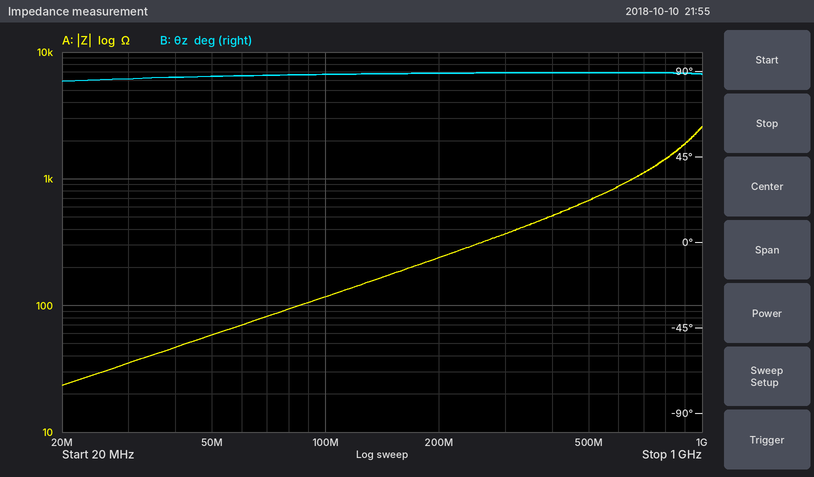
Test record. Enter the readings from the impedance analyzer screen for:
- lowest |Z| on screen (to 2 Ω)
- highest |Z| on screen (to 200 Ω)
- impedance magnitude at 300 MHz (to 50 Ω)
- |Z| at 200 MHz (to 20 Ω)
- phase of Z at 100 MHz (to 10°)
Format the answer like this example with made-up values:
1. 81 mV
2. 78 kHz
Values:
1. 24 Ω
2. 2.6 kΩ
3. 350 Ω
4. 240 Ω
5. 90°
